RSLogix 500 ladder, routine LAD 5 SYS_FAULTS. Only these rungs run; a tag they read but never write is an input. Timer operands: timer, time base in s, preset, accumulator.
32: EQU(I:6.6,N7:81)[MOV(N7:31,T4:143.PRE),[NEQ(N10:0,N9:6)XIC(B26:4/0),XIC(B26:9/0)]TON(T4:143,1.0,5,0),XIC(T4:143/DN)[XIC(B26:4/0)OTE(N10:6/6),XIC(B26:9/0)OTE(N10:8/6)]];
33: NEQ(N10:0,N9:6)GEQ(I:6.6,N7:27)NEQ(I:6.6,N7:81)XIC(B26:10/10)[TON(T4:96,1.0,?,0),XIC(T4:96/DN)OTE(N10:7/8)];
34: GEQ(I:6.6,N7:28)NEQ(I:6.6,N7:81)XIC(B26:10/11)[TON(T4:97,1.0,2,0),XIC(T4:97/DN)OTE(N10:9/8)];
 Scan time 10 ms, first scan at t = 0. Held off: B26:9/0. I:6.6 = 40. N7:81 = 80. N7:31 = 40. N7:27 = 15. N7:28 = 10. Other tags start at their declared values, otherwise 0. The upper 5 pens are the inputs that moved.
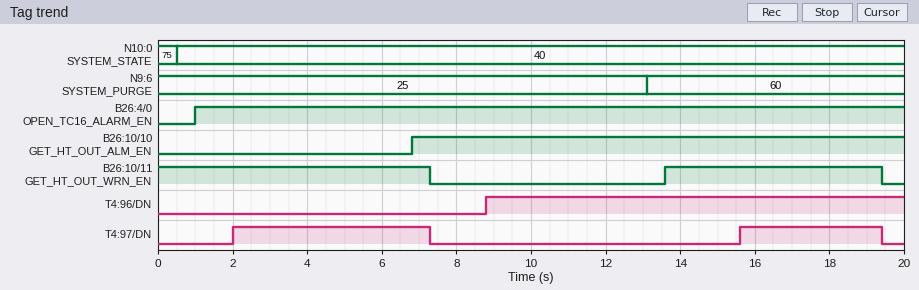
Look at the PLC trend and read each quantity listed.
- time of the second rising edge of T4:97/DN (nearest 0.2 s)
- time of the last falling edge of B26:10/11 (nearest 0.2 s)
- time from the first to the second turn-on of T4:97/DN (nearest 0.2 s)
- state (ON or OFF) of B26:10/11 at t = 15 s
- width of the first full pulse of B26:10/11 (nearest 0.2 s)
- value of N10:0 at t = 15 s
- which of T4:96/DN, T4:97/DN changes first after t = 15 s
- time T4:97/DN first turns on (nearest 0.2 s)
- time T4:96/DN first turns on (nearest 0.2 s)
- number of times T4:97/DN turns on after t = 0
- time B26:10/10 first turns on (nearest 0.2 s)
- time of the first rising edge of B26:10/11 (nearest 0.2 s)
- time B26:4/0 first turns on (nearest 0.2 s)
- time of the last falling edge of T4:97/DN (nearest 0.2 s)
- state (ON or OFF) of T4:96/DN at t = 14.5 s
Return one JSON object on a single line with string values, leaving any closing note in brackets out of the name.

{"time of the second rising edge of T4:97/DN": "15.6 s", "time of the last falling edge of B26:10/11": "19.4 s", "time from the first to the second turn-on of T4:97/DN": "13.6 s", "state (ON or OFF) of B26:10/11 at t = 15 s": "ON", "width of the first full pulse of B26:10/11": "5.8 s", "value of N10:0 at t = 15 s": "40", "which of T4:96/DN, T4:97/DN changes first after t = 15 s": "T4:97/DN", "time T4:97/DN first turns on": "2.0 s", "time T4:96/DN first turns on": "8.8 s", "number of times T4:97/DN turns on after t = 0": "2", "time B26:10/10 first turns on": "6.8 s", "time of the first rising edge of B26:10/11": "13.6 s", "time B26:4/0 first turns on": "1.0 s", "time of the last falling edge of T4:97/DN": "19.4 s", "state (ON or OFF) of T4:96/DN at t = 14.5 s": "ON"}
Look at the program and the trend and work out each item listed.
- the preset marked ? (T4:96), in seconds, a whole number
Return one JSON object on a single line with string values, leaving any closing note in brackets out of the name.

{"the preset marked ? (T4:96), in seconds, a whole number": "2 s"}
